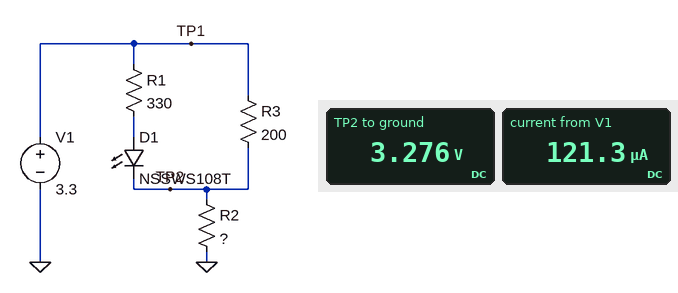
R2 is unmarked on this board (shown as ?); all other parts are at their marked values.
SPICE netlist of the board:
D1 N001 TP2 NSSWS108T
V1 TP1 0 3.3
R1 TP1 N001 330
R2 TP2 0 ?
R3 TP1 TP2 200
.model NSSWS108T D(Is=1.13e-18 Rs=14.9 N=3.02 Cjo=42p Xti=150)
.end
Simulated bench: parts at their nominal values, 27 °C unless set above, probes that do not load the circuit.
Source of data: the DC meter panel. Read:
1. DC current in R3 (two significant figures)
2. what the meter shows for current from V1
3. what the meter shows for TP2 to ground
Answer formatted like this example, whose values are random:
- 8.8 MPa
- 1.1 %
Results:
- 120 µA
- 121.3 µA
- 3.276 V
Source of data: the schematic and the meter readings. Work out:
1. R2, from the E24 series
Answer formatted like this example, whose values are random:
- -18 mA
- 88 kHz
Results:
- 27 kΩ
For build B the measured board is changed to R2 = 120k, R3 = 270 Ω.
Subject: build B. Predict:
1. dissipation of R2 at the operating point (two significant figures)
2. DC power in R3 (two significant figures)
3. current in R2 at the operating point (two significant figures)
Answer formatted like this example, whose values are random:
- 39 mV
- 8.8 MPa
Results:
- 90 µW
- 200 nW
- 27 µA
